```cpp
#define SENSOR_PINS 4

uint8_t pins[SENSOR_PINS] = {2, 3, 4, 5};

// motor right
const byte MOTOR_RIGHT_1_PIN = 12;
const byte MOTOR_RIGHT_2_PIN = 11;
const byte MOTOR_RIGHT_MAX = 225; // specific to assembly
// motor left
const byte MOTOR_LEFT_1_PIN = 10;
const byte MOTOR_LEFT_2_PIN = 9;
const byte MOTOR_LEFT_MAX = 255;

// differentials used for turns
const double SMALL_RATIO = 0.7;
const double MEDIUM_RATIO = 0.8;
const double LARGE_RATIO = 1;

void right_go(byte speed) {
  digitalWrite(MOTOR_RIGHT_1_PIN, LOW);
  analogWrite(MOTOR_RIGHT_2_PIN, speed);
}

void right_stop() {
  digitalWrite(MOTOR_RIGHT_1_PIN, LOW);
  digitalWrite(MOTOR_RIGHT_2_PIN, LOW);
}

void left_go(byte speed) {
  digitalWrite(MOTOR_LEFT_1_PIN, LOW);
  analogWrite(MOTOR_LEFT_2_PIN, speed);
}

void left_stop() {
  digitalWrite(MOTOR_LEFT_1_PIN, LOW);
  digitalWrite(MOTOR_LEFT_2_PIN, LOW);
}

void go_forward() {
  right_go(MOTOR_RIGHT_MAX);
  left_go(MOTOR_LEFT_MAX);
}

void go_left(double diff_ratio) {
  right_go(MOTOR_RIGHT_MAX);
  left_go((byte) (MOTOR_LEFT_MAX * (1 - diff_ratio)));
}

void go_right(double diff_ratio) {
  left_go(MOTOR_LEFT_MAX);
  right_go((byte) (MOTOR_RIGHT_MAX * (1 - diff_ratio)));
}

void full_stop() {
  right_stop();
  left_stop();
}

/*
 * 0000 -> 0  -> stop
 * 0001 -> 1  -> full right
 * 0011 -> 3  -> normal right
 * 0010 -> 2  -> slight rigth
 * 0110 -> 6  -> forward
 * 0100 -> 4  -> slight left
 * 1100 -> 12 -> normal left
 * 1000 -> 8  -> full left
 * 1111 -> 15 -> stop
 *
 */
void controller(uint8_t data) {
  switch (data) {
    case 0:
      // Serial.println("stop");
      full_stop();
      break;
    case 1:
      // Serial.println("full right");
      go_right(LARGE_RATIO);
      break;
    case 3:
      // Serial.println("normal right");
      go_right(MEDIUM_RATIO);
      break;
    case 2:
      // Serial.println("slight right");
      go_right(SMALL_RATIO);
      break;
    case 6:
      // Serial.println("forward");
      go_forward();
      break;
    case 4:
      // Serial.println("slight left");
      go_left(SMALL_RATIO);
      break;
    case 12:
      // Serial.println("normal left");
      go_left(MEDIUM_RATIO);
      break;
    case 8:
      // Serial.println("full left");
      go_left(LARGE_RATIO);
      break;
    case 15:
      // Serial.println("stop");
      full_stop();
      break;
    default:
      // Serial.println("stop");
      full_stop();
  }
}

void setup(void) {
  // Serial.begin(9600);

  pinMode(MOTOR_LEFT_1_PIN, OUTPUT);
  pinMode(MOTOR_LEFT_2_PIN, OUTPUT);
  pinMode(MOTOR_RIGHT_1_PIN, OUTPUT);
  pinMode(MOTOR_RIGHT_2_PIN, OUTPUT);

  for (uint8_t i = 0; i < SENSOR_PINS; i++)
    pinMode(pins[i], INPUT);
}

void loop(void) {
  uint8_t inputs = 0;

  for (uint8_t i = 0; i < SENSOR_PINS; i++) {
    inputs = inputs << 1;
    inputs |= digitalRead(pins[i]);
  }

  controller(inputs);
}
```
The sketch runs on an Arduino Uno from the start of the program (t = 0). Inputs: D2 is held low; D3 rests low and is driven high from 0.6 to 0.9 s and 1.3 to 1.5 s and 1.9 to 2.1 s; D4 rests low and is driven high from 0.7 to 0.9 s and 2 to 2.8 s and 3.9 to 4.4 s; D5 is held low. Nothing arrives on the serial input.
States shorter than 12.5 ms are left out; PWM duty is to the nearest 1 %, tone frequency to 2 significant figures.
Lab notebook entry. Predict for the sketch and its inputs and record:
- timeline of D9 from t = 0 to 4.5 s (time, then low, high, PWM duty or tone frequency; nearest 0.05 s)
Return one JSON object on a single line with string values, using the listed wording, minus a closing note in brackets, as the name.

{"timeline of D9 from t = 0 to 4.5 s": "0 s low; 0.6 s PWM 30 %; 0.7 s high; 0.9 s low; 1.3 s PWM 30 %; 1.5 s low; 1.9 s PWM 30 %; 2 s high; 2.8 s low; 3.9 s high; 4.4 s low"}
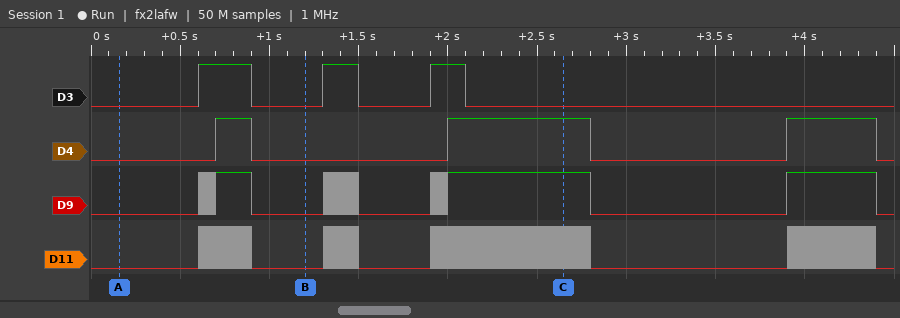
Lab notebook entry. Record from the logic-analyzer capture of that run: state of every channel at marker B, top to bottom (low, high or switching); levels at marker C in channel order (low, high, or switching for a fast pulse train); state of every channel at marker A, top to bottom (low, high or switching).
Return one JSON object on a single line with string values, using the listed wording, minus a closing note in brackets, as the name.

{"state of every channel at marker B, top to bottom": "D3 low, D4 low, D9 low, D11 low", "levels at marker C in channel order": "D3 low, D4 high, D9 high, D11 switching", "state of every channel at marker A, top to bottom": "D3 low, D4 low, D9 low, D11 low"}
